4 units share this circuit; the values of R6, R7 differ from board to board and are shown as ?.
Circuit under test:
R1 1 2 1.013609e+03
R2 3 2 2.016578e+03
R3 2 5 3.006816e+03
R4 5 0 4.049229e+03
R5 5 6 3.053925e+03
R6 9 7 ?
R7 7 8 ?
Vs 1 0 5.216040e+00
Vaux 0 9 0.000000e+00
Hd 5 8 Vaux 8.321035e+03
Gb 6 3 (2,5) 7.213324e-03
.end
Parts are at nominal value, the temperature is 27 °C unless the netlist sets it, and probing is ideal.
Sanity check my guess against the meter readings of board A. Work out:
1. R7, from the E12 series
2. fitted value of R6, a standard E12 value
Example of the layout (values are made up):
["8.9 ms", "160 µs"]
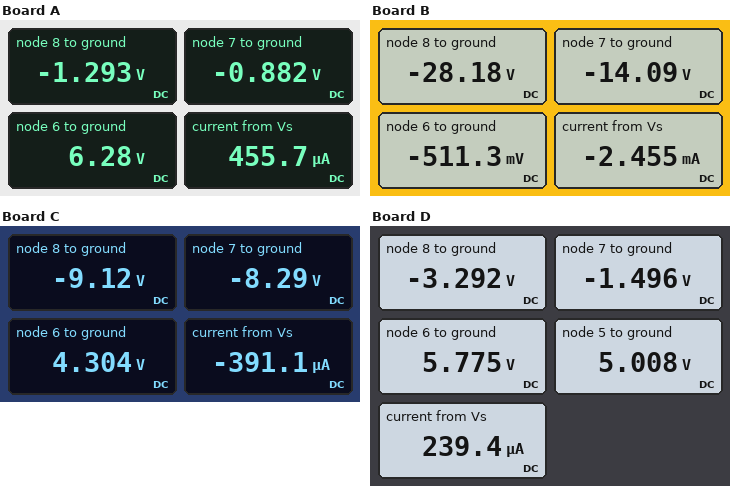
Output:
["560 Ω", "1.2 kΩ"]
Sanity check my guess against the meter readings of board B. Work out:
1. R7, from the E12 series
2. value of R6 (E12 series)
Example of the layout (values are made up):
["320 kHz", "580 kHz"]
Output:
["3.3 kΩ", "3.3 kΩ"]
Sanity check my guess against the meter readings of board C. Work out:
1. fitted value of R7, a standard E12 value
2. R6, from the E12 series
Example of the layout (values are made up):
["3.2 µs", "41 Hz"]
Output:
["470 Ω", "4.7 kΩ"]
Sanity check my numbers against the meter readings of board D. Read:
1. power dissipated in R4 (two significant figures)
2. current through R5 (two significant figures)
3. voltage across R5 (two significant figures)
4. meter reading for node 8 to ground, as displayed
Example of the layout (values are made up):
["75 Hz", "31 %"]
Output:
["6.2 mW", "250 µA", "770 mV", "-3.292 V"]
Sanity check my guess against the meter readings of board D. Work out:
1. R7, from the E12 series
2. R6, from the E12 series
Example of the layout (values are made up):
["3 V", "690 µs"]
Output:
["1.8 kΩ", "1.5 kΩ"]
